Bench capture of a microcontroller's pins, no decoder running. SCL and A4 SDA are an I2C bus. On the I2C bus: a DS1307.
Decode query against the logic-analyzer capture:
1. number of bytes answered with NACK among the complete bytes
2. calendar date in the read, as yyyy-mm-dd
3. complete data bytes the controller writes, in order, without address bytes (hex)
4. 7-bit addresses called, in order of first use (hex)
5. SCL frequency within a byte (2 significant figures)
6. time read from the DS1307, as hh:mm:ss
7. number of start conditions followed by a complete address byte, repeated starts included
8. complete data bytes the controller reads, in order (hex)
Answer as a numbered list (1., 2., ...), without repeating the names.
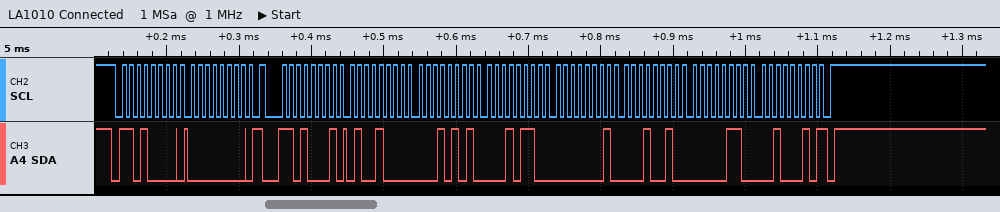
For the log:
1. 1
2. 2022-06-12
3. 00
4. 0x68
5. 100 kHz
6. 16:15:48
7. 2
8. 48 15 16 01 12 06 22
